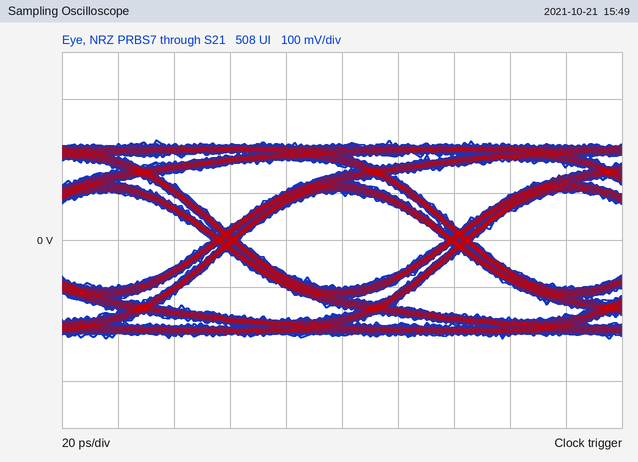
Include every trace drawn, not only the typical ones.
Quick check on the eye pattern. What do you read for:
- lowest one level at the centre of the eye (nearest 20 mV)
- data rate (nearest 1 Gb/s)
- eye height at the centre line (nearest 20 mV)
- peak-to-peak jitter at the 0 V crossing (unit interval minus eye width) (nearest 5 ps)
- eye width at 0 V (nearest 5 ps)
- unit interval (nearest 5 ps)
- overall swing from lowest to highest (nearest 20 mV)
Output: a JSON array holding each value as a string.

["100 mV", "12 Gb/s", "200 mV", "10 ps", "75 ps", "85 ps", "420 mV"]
